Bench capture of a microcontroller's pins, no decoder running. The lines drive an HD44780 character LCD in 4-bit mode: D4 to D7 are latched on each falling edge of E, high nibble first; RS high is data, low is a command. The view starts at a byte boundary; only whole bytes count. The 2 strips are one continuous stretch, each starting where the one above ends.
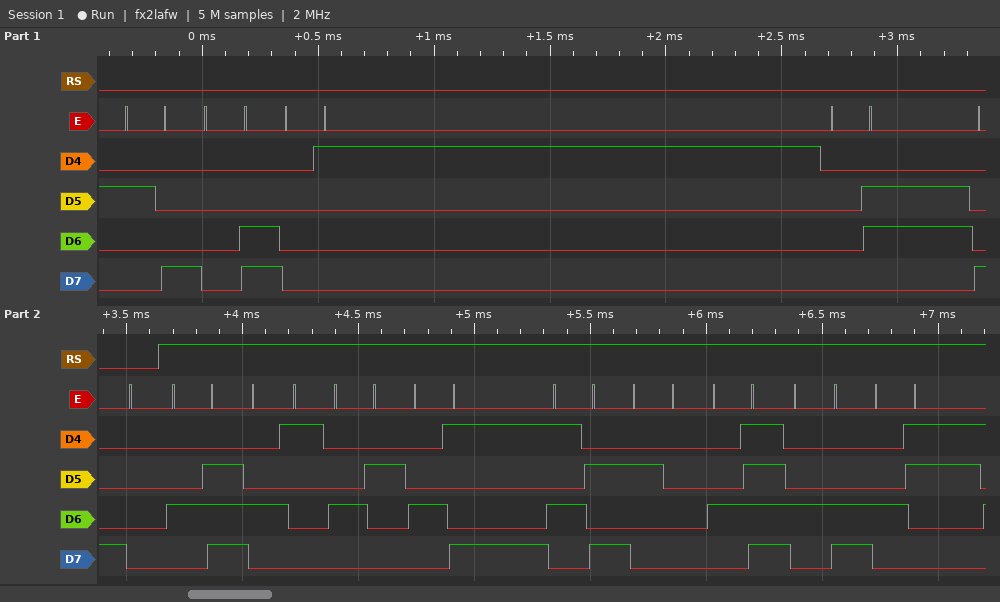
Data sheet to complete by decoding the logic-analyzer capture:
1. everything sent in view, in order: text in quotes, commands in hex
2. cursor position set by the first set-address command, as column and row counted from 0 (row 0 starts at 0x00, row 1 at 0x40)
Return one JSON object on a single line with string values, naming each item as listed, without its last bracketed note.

{"everything sent in view, in order: text in quotes, commands in hex": "0x28 0x0C 0x01 0x06 0x80 \"NABIZ OLC\"", "cursor position set by the first set-address command, as column and row counted from 0": "column 0, row 0"}
